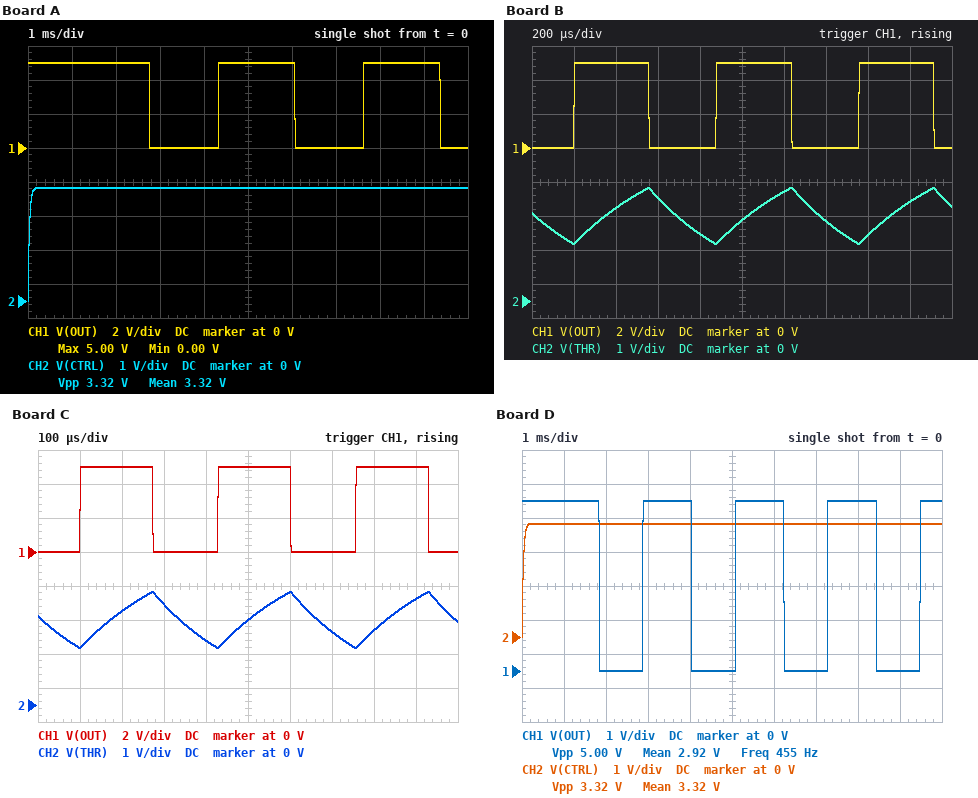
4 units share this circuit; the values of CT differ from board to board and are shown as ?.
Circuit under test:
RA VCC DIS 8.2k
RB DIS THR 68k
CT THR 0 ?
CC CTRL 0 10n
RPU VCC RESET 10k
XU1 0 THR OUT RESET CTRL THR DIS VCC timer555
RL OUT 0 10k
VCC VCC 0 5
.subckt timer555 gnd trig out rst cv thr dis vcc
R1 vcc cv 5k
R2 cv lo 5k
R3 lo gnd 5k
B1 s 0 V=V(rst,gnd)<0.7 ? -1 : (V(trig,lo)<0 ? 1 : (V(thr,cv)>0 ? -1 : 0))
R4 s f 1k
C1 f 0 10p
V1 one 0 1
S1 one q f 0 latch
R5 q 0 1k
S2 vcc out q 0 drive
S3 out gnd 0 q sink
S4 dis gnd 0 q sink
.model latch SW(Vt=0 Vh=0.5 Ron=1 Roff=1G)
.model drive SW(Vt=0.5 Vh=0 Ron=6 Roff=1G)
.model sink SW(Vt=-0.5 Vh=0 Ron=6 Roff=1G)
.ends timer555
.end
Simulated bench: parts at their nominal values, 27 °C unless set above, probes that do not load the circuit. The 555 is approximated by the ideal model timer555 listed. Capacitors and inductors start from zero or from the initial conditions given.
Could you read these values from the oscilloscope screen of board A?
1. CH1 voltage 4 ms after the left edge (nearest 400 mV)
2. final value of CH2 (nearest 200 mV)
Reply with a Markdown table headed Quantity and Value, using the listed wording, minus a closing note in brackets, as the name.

| Quantity | Value |
|---|---|
| CH1 voltage 4 ms after the left edge | 0 V |
| final value of CH2 | 3.4 V |
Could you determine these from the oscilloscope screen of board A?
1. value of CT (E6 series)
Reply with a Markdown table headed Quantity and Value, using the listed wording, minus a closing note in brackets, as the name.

| Quantity | Value |
|---|---|
| value of CT | 33 nF |
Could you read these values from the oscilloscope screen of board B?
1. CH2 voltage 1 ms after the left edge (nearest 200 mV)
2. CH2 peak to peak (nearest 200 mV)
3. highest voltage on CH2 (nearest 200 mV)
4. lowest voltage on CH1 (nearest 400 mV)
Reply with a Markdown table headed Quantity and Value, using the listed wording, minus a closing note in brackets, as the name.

| Quantity | Value |
|---|---|
| CH2 voltage 1 ms after the left edge | 2.4 V |
| CH2 peak to peak | 1.6 V |
| highest voltage on CH2 | 3.4 V |
| lowest voltage on CH1 | 0 V |
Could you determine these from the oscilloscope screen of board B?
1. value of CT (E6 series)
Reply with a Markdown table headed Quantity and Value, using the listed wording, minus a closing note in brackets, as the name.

| Quantity | Value |
|---|---|
| value of CT | 6.8 nF |
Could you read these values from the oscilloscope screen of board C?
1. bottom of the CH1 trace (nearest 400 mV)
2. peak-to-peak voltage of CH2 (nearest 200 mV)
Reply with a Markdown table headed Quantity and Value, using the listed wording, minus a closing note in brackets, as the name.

| Quantity | Value |
|---|---|
| bottom of the CH1 trace | 0 V |
| peak-to-peak voltage of CH2 | 1.6 V |
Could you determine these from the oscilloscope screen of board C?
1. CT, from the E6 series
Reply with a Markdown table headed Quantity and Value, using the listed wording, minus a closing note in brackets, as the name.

| Quantity | Value |
|---|---|
| CT, from the E6 series | 3.3 nF |
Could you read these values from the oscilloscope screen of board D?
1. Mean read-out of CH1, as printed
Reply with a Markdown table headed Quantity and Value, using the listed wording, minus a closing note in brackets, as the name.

| Quantity | Value |
|---|---|
| Mean read-out of CH1, as printed | 2.92 V |
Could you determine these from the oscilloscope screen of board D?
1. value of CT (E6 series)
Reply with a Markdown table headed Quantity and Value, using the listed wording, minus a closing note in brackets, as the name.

| Quantity | Value |
|---|---|
| value of CT | 22 nF |
